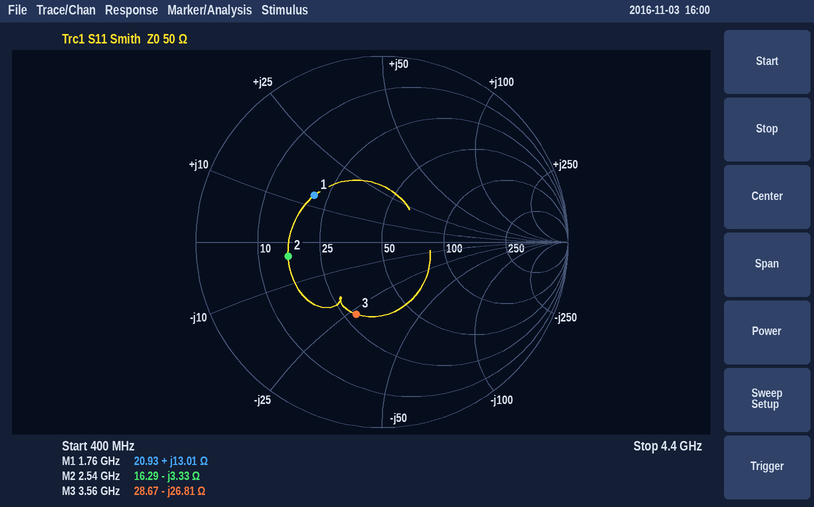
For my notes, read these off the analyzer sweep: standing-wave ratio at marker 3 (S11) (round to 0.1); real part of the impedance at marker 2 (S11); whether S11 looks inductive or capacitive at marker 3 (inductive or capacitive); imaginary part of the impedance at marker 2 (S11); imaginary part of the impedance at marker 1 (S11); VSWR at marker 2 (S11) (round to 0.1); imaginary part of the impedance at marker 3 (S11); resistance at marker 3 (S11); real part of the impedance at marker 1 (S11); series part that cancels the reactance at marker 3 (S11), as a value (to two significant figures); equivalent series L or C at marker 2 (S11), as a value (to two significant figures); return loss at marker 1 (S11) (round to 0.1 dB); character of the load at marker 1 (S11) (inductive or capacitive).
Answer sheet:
2.4
16.29 Ω
capacitive
-3.33 Ω
+13.01 Ω
3.1
-26.81 Ω
28.67 Ω
20.93 Ω
1.2 nH
19 pF
7.1 dB
inductive
